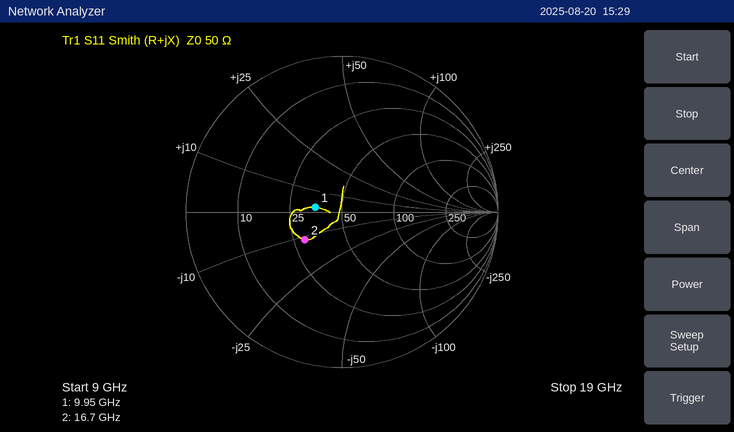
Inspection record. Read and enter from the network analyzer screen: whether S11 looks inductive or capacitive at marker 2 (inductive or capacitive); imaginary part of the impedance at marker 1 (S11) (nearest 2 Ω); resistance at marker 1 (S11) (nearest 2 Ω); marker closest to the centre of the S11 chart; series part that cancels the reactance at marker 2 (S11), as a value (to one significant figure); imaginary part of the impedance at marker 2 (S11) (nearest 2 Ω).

capacitive
+2 Ω
36 Ω
marker 1
100 pH
-12 Ω
